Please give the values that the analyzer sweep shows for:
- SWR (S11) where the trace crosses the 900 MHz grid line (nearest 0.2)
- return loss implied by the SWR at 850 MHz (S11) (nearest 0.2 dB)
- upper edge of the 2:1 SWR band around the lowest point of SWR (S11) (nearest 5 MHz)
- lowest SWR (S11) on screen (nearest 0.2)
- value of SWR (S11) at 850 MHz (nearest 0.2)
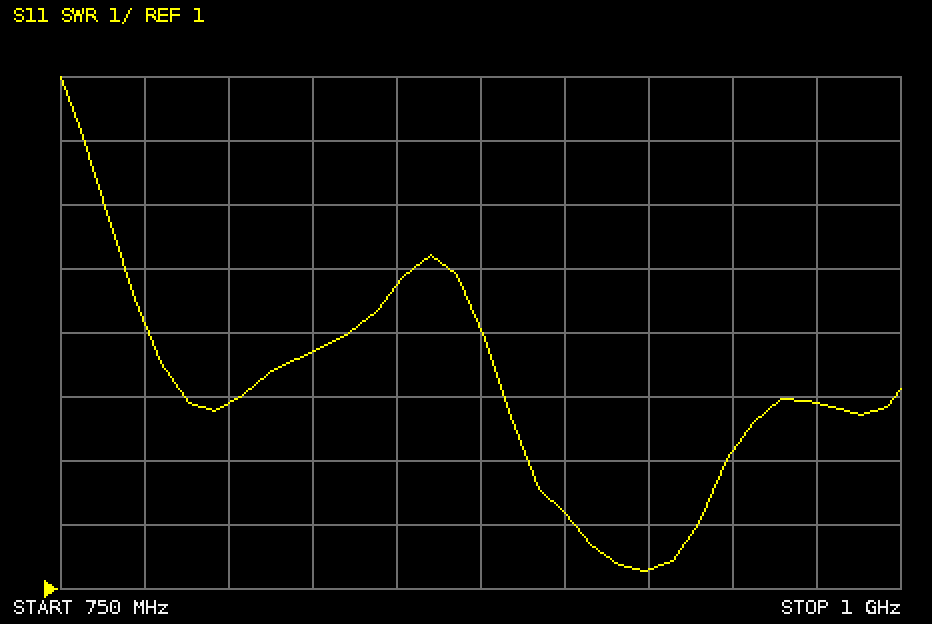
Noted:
2.2
3.0 dB
940 MHz
1.2
5.8
